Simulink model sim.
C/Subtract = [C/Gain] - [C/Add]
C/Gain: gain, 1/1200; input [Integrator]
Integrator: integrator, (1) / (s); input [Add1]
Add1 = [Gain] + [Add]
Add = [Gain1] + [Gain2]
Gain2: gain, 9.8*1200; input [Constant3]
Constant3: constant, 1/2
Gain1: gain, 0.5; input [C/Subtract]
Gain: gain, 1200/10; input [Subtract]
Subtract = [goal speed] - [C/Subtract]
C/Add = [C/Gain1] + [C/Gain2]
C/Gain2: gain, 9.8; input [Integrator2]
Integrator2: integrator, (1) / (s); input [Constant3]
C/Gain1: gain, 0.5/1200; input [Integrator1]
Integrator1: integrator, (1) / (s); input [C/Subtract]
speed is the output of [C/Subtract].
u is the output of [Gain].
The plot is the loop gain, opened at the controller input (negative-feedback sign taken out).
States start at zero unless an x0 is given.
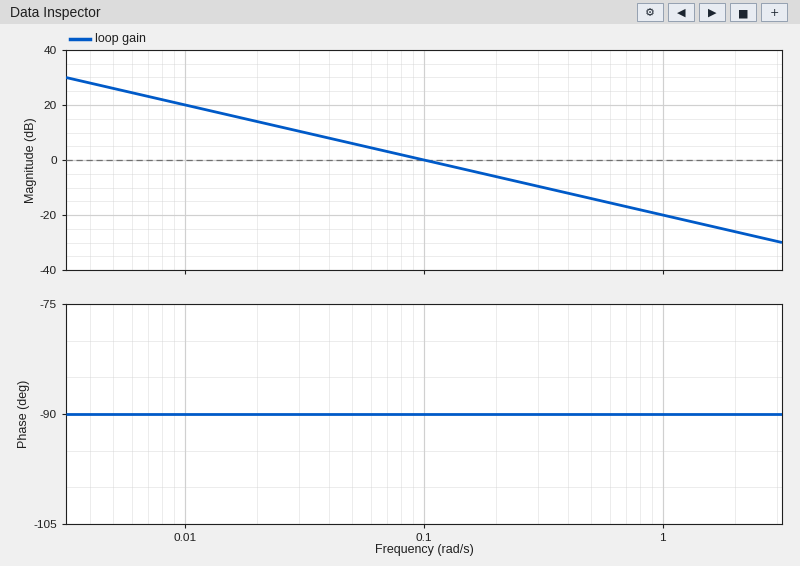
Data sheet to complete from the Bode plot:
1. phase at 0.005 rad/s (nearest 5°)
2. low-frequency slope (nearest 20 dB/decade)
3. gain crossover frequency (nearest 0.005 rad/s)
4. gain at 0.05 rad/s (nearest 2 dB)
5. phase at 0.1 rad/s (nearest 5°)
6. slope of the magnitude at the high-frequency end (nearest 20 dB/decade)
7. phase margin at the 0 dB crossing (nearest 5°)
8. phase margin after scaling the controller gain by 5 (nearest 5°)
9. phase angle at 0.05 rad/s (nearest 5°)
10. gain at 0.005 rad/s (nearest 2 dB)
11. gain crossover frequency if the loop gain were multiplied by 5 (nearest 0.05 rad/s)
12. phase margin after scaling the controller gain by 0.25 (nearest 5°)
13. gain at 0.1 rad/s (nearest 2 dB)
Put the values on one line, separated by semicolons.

-90°; -20 dB/decade; 0.100 rad/s; 6 dB; -90°; -20 dB/decade; 90°; 90°; -90°; 26 dB; 0.50 rad/s; 90°; 0 dB
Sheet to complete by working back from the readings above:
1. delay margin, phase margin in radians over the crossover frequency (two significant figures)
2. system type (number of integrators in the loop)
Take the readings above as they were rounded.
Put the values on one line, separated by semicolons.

16 s; 1
